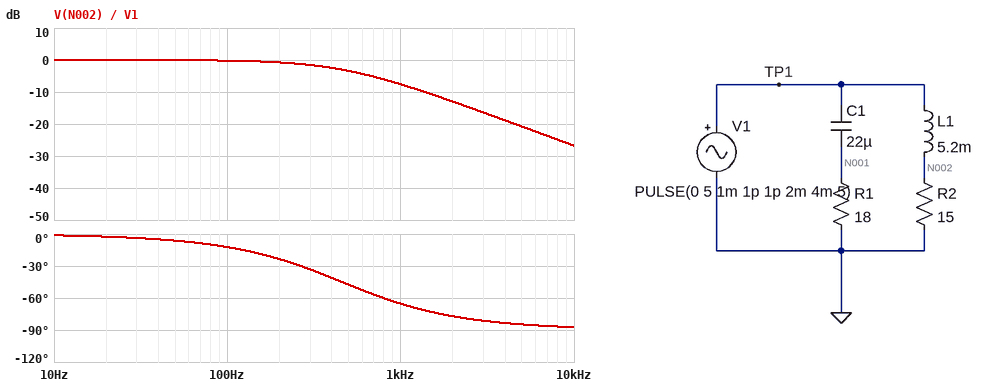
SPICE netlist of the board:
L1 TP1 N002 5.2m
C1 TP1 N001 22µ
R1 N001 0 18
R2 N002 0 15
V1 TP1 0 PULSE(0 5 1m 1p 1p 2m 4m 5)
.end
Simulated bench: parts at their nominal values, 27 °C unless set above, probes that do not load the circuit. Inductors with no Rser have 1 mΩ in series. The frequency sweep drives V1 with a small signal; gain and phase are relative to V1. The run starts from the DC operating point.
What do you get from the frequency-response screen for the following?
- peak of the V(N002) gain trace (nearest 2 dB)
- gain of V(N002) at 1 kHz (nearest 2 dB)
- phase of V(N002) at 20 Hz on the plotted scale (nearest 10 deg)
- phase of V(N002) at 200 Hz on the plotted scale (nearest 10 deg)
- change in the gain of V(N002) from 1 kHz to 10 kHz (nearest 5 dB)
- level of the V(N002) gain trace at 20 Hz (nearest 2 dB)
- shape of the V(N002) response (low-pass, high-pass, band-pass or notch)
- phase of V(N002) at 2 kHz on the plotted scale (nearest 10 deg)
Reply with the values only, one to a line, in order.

0 dB
-8 dB
0 deg
-20 deg
-20 dB
0 dB
low-pass
-80 deg
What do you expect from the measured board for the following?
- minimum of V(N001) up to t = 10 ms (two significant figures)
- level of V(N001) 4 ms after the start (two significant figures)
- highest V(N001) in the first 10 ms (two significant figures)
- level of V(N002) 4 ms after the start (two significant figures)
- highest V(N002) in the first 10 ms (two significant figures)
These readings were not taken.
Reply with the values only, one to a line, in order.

-5.0 V
-400 mV
5.0 V
280 mV
5.0 V
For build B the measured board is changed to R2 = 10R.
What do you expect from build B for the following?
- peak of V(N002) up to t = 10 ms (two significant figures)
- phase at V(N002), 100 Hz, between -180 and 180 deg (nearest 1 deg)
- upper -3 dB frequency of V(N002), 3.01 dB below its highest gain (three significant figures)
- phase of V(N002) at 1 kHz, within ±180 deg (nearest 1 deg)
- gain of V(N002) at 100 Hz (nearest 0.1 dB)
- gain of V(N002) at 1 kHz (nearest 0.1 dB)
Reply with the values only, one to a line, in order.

4.9 V
-18 deg
306 Hz
-73 deg
-0.4 dB
-10.7 dB
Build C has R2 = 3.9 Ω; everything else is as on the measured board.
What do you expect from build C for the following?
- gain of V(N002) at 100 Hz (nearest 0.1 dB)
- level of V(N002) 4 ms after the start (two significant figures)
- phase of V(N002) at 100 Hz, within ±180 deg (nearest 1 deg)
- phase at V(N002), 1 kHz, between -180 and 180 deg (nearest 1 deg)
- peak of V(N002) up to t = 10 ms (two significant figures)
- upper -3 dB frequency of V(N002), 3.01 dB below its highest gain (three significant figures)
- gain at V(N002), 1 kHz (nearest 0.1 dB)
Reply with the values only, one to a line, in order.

-2.3 dB
1.8 V
-40 deg
-83 deg
4.1 V
119 Hz
-18.5 dB
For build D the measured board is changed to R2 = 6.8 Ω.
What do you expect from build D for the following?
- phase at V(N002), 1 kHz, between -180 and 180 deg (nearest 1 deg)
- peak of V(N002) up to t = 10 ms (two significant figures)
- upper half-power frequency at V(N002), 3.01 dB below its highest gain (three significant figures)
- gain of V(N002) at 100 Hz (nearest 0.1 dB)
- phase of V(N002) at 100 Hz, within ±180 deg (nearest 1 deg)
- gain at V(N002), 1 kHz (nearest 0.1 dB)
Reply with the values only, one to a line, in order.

-78 deg
4.7 V
208 Hz
-0.9 dB
-26 deg
-13.8 dB
